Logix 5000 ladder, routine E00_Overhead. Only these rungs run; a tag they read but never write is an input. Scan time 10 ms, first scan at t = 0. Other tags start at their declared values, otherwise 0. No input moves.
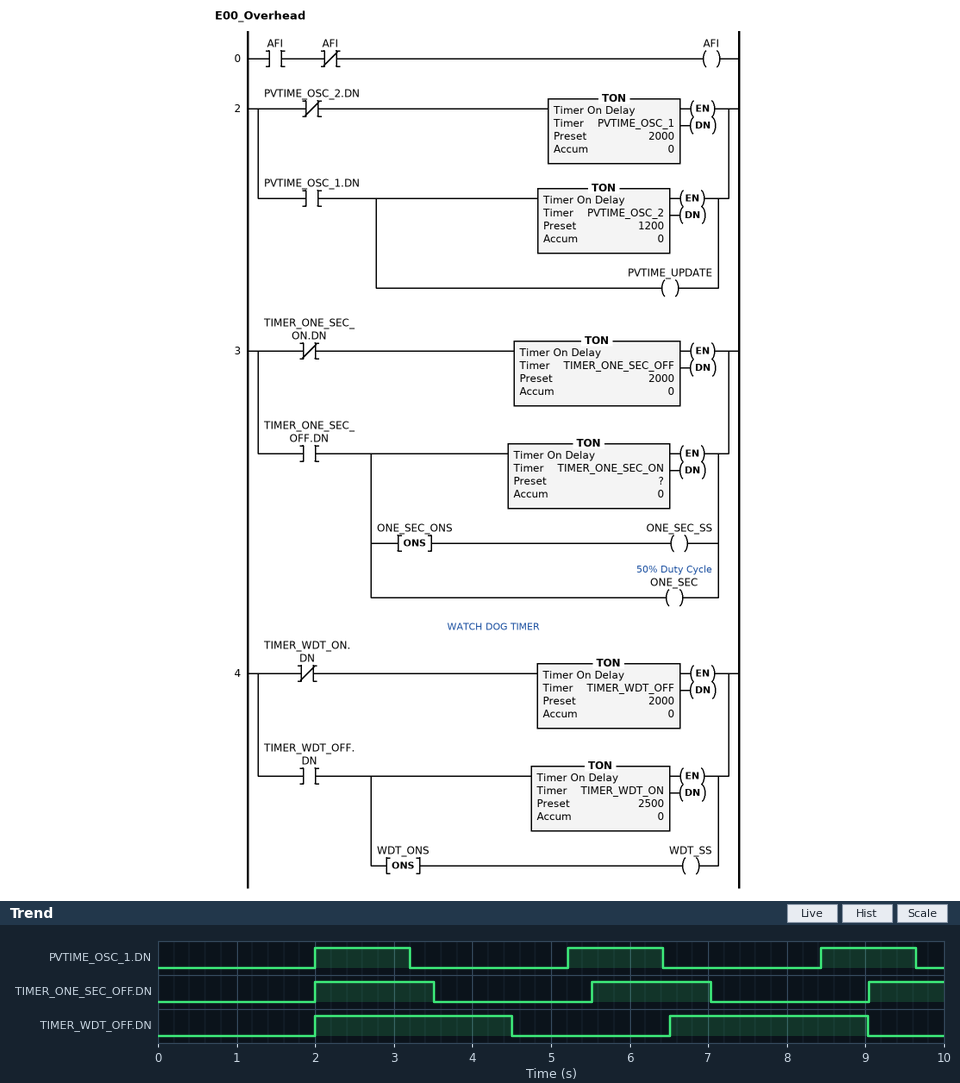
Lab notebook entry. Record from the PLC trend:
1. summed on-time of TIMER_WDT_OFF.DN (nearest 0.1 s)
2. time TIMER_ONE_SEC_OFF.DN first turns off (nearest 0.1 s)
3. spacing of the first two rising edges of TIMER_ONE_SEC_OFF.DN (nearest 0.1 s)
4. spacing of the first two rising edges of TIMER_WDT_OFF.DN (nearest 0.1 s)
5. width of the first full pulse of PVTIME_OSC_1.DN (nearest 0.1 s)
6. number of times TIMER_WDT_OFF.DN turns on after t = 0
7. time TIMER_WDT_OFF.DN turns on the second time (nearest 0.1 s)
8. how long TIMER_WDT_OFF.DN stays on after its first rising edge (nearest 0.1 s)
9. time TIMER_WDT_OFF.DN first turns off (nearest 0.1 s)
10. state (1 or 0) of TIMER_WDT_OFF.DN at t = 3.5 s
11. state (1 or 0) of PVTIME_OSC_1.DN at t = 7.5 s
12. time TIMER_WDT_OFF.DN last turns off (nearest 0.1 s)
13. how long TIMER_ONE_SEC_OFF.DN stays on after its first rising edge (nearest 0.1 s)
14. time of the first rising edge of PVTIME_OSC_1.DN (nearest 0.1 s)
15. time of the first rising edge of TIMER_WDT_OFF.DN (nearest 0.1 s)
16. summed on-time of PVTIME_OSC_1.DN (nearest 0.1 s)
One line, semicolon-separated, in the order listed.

5.0 s; 3.5 s; 3.5 s; 4.5 s; 1.2 s; 2; 6.5 s; 2.5 s; 4.5 s; 1; 0; 9.0 s; 1.5 s; 2.0 s; 2.0 s; 3.6 s
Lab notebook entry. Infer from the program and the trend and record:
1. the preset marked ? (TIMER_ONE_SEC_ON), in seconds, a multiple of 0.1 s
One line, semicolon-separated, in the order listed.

1.5 s
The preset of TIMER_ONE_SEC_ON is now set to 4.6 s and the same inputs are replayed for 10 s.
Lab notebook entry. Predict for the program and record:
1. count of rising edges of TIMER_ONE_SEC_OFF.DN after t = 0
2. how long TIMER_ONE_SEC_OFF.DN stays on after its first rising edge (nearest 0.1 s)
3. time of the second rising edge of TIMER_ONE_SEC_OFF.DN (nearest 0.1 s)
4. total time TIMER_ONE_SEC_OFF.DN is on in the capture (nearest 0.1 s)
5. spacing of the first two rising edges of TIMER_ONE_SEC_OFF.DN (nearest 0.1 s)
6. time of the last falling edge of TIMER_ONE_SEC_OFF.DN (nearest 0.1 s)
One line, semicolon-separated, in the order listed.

2; 4.6 s; 8.6 s; 6.0 s; 6.6 s; 6.6 s
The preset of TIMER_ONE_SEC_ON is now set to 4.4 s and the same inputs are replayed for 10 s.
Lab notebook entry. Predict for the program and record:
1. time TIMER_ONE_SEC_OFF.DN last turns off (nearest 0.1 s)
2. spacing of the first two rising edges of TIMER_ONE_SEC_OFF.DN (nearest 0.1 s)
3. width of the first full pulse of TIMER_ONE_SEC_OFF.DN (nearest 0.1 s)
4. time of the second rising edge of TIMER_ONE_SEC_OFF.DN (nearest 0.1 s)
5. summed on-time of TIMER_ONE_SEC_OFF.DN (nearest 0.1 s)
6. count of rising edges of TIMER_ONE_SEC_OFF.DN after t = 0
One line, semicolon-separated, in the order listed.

6.4 s; 6.4 s; 4.4 s; 8.4 s; 6.0 s; 2
